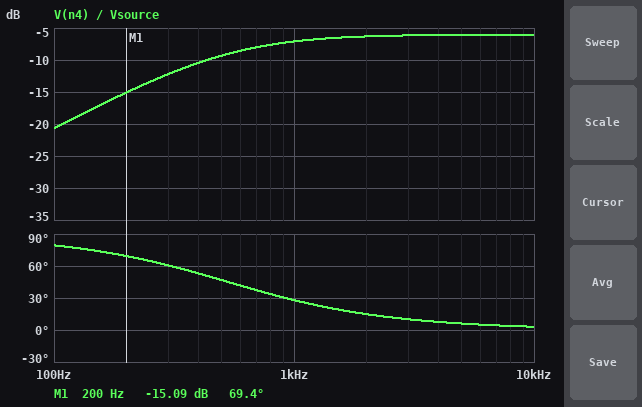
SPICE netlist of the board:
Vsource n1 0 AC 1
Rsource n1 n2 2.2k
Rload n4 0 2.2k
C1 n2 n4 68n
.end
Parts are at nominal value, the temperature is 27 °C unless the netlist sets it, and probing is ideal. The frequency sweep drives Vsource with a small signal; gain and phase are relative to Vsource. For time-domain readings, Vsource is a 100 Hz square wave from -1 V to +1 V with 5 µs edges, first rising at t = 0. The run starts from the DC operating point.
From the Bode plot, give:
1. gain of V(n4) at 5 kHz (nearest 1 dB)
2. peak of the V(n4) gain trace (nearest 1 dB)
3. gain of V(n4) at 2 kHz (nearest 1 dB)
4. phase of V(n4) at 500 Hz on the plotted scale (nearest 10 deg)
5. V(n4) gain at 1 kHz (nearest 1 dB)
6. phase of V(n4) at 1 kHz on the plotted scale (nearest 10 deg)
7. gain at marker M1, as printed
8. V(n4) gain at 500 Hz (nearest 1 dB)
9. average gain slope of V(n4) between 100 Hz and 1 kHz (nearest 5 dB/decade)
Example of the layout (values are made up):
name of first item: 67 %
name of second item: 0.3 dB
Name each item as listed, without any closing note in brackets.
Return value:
gain of V(n4) at 5 kHz: -6 dB
peak of the V(n4) gain trace: -6 dB
gain of V(n4) at 2 kHz: -6 dB
phase of V(n4) at 500 Hz on the plotted scale: 50 deg
V(n4) gain at 1 kHz: -7 dB
phase of V(n4) at 1 kHz on the plotted scale: 30 deg
gain at marker M1, as printed: -15.09 dB
V(n4) gain at 500 Hz: -9 dB
average gain slope of V(n4) between 100 Hz and 1 kHz: 15 dB/decade
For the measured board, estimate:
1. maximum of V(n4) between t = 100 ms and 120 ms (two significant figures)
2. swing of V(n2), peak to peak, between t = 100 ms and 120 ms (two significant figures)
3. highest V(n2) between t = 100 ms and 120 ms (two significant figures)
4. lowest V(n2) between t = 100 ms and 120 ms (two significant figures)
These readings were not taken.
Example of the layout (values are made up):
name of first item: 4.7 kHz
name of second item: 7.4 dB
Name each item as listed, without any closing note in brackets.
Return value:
maximum of V(n4) between t = 100 ms and 120 ms: 990 mV
swing of V(n2), peak to peak, between t = 100 ms and 120 ms: 2.0 V
highest V(n2) between t = 100 ms and 120 ms: 1.0 V
lowest V(n2) between t = 100 ms and 120 ms: -1.0 V
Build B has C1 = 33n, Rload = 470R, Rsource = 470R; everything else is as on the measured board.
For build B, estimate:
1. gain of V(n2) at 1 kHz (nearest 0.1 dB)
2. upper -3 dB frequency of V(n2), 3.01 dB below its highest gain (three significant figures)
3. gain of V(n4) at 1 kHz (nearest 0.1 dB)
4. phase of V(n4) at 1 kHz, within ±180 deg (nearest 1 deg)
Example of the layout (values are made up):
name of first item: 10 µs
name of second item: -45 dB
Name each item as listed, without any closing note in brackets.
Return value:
gain of V(n2) at 1 kHz: -0.1 dB
upper -3 dB frequency of V(n2), 3.01 dB below its highest gain: 7.26 kHz
gain of V(n4) at 1 kHz: -20.4 dB
phase of V(n4) at 1 kHz, within ±180 deg: 79 deg
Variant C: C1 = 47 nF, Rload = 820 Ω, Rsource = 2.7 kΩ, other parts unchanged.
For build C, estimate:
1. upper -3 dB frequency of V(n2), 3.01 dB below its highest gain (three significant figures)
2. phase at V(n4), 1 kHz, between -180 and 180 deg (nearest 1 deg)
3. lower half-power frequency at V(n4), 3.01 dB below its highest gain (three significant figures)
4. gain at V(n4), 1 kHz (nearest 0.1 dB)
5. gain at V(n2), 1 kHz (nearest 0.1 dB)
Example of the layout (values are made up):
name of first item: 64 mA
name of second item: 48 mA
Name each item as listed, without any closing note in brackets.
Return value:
upper -3 dB frequency of V(n2), 3.01 dB below its highest gain: 1.02 kHz
phase at V(n4), 1 kHz, between -180 and 180 deg: 44 deg
lower half-power frequency at V(n4), 3.01 dB below its highest gain: 962 Hz
gain at V(n4), 1 kHz: -15.5 dB
gain at V(n2), 1 kHz: -2.9 dB
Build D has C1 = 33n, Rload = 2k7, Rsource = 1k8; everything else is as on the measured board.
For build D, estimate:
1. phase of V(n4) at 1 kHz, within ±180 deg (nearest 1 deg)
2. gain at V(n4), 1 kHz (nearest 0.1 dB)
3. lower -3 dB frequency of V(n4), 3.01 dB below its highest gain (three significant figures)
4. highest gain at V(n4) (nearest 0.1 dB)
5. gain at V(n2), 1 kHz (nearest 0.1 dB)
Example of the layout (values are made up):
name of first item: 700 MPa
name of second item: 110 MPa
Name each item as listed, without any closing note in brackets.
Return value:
phase of V(n4) at 1 kHz, within ±180 deg: 47 deg
gain at V(n4), 1 kHz: -7.8 dB
lower -3 dB frequency of V(n4), 3.01 dB below its highest gain: 1.07 kHz
highest gain at V(n4): -4.4 dB
gain at V(n2), 1 kHz: -1.5 dB
